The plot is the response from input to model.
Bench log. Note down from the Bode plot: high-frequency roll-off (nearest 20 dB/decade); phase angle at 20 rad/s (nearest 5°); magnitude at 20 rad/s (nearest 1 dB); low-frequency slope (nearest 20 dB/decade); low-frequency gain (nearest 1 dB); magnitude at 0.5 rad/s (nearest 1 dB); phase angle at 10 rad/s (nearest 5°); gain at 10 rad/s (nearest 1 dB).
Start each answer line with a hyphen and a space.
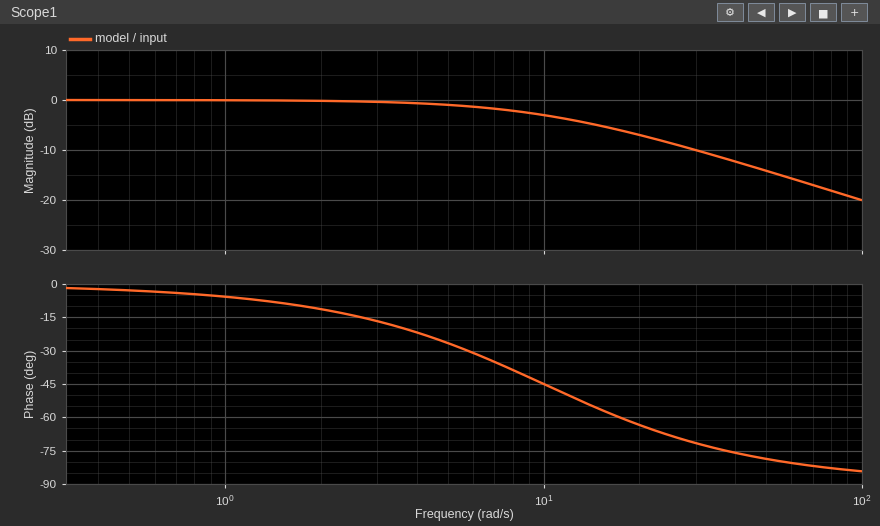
- -20 dB/decade
- -65°
- -7 dB
- 0 dB/decade
- 0 dB
- 0 dB
- -45°
- -3 dB
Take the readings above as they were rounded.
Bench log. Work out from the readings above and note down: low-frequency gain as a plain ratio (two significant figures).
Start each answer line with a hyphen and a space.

- 1.0
